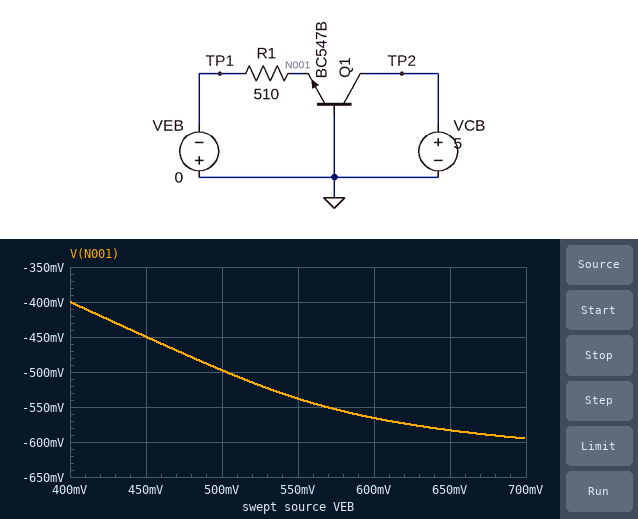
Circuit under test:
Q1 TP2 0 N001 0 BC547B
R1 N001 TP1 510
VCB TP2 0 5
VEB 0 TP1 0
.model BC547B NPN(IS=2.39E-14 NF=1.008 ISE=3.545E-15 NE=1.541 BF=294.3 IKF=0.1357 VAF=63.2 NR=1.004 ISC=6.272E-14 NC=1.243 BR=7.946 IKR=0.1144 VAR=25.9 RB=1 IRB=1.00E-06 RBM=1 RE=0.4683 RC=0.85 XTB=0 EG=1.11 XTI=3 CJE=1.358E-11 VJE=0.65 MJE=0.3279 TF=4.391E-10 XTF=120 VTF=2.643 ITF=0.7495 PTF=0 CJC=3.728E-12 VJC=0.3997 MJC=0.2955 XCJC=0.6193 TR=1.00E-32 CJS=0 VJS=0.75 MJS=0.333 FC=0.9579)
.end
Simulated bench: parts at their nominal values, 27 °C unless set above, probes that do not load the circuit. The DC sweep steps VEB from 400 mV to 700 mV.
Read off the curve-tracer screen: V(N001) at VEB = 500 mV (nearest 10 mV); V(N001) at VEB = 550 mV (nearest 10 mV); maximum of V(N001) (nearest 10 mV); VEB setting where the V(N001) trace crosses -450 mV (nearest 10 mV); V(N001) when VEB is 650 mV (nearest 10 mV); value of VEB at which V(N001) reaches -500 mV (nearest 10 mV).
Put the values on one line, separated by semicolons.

-500 mV; -540 mV; -400 mV; 450 mV; -580 mV; 500 mV
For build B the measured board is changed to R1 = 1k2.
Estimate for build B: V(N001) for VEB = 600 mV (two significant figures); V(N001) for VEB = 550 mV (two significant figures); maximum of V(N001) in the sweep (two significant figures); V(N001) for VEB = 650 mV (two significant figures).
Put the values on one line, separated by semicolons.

-550 mV; -530 mV; -400 mV; -570 mV
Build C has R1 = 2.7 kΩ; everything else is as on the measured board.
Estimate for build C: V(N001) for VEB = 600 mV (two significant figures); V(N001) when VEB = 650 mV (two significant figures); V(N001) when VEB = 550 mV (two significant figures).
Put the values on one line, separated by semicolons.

-540 mV; -550 mV; -520 mV
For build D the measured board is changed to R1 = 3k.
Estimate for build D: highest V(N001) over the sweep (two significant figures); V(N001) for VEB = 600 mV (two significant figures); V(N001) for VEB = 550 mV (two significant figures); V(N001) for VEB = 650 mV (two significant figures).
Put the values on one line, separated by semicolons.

-400 mV; -540 mV; -520 mV; -550 mV
